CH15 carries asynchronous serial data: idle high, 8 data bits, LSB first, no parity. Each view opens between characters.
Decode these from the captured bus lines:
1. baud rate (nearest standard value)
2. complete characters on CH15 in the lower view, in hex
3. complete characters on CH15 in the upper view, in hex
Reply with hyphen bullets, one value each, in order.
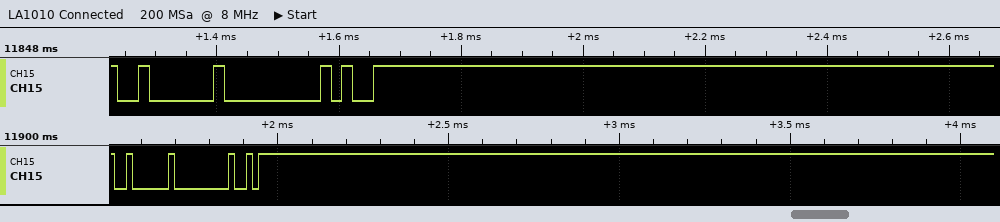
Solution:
- 57600 baud
- 02, 00, FA
- 02, 00, F9
